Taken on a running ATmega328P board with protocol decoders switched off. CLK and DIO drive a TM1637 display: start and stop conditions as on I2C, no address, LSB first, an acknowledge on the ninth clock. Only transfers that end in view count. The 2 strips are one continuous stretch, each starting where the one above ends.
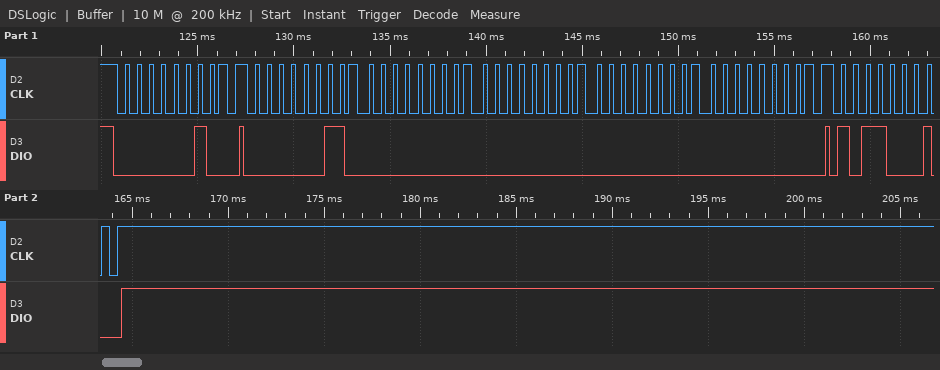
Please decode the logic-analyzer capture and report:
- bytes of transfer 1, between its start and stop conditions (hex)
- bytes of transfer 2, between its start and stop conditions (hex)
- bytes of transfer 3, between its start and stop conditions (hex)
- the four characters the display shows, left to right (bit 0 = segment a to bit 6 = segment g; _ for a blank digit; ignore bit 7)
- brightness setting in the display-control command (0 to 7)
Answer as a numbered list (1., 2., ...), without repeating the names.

1. 40
2. C0 00 00 00 00
3. 8D
4. ____
5. 5
